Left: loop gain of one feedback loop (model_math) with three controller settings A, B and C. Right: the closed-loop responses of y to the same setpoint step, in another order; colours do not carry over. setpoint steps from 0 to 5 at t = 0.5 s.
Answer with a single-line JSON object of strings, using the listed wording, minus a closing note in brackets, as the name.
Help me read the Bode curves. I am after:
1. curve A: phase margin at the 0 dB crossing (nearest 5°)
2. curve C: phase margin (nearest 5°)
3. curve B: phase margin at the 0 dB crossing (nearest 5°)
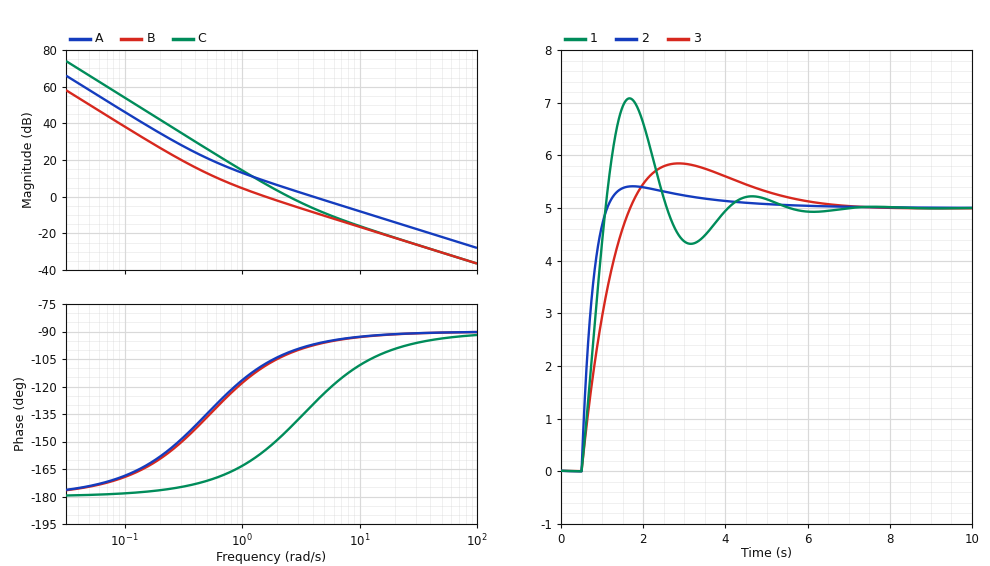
{"curve A: phase margin at the 0 dB crossing": "85°", "curve C: phase margin": "35°", "curve B: phase margin at the 0 dB crossing": "70°"}
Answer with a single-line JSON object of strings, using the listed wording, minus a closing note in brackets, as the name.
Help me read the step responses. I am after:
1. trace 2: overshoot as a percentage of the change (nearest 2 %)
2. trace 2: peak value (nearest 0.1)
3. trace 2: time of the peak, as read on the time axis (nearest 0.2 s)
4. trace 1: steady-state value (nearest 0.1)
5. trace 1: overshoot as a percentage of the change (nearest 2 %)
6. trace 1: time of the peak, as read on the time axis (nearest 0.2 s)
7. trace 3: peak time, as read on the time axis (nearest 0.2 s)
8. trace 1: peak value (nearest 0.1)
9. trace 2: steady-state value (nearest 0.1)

{"trace 2: overshoot as a percentage of the change": "8 %", "trace 2: peak value": "5.4", "trace 2: time of the peak, as read on the time axis": "1.8 s", "trace 1: steady-state value": "5.0", "trace 1: overshoot as a percentage of the change": "42 %", "trace 1: time of the peak, as read on the time axis": "1.6 s", "trace 3: peak time, as read on the time axis": "2.8 s", "trace 1: peak value": "7.1", "trace 2: steady-state value": "5.0"}
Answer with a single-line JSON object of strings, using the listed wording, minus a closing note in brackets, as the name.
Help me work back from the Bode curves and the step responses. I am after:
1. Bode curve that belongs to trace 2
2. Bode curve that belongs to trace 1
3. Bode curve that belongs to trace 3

{"Bode curve that belongs to trace 2": "A", "Bode curve that belongs to trace 1": "C", "Bode curve that belongs to trace 3": "B"}
